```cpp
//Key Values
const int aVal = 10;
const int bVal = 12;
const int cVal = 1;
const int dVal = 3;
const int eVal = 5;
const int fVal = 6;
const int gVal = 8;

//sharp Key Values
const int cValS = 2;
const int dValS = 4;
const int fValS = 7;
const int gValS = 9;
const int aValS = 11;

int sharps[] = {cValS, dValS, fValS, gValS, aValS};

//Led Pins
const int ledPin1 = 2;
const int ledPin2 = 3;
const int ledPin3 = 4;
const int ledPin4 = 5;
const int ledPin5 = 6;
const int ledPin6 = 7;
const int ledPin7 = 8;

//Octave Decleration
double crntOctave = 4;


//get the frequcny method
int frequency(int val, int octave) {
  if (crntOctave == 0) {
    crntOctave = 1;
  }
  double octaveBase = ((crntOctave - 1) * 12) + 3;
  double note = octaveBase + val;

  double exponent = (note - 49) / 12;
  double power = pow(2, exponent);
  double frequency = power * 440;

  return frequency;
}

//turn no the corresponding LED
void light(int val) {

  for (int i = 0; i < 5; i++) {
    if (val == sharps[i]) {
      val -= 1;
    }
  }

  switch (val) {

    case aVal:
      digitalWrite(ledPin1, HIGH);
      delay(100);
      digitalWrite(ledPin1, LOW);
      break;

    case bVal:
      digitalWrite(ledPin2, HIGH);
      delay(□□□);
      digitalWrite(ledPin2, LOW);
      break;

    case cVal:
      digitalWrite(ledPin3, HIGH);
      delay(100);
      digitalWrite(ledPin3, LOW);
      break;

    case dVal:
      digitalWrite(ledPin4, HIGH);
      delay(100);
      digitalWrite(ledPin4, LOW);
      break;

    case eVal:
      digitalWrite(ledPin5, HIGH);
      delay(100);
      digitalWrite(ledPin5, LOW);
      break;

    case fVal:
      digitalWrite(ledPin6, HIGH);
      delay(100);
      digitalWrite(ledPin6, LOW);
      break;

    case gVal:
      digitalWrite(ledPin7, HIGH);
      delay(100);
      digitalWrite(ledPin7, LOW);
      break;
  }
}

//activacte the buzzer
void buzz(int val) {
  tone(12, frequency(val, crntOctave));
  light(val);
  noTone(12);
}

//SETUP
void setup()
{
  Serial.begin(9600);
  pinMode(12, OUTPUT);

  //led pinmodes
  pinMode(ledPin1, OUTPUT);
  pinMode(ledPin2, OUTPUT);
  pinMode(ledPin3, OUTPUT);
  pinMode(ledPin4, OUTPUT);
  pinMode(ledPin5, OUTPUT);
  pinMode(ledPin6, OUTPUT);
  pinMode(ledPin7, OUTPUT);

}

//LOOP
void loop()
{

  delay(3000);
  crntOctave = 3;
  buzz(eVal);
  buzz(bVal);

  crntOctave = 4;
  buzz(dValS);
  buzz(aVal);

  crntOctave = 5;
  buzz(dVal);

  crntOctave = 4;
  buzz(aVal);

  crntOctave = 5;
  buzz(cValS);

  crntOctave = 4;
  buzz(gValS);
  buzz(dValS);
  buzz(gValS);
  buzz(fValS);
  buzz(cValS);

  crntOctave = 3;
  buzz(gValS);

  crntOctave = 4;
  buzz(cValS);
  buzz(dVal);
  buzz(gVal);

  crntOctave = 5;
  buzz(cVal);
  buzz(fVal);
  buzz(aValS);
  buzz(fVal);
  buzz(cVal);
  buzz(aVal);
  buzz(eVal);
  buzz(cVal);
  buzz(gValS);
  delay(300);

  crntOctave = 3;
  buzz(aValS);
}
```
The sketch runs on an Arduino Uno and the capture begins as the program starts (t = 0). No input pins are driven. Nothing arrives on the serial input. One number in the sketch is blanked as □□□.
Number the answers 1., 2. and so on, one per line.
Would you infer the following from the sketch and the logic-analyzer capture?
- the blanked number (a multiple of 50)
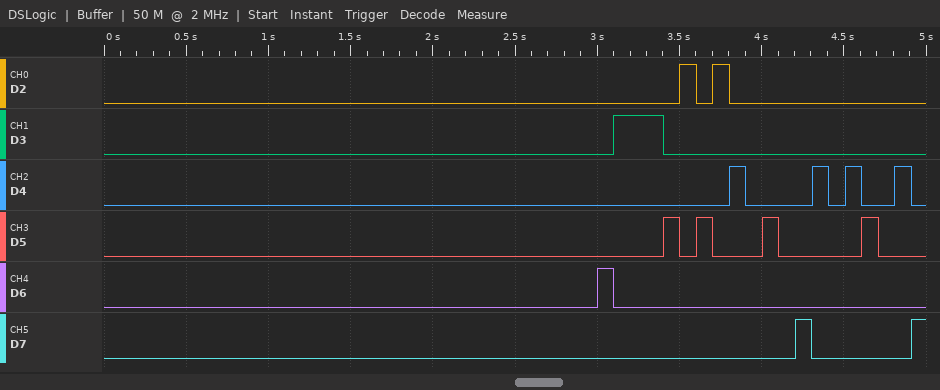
1. 300
